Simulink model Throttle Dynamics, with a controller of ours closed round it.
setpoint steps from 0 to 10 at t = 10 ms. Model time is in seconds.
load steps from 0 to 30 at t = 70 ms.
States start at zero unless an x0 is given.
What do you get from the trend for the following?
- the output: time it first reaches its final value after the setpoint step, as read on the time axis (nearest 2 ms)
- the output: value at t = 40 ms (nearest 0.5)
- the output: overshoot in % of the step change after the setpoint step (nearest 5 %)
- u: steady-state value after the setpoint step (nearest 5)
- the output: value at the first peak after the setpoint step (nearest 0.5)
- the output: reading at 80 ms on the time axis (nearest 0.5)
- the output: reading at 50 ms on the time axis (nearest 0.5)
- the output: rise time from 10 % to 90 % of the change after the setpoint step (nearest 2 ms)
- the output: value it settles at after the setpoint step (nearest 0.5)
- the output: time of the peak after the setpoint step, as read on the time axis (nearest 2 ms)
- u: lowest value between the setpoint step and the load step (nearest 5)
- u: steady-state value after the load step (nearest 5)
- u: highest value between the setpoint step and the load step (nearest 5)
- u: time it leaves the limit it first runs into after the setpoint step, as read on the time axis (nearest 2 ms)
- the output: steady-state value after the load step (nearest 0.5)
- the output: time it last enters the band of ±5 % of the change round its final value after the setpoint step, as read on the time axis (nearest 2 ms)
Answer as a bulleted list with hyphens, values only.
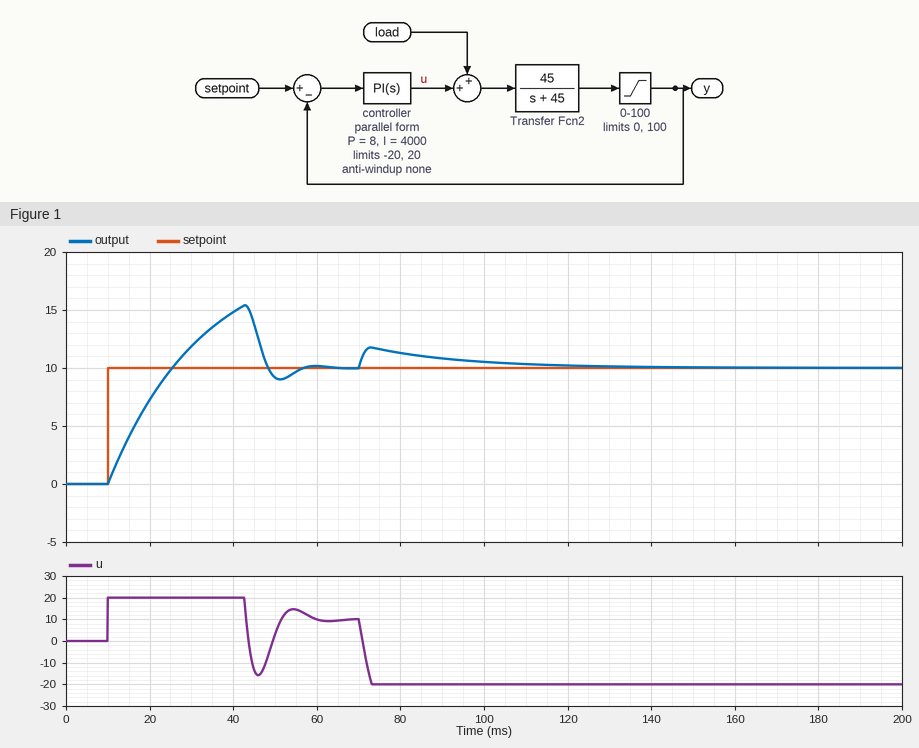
- 26 ms
- 15.0
- 55 %
- 10
- 15.5
- 11.5
- 9.0
- 12 ms
- 10.0
- 42 ms
- -15
- -20
- 20
- 42 ms
- 10.0
- 54 ms
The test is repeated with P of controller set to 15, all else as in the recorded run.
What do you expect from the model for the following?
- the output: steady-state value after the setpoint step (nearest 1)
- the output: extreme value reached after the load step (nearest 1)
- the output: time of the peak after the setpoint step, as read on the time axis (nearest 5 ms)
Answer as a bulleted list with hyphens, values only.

- 10
- 11
- 40 ms
